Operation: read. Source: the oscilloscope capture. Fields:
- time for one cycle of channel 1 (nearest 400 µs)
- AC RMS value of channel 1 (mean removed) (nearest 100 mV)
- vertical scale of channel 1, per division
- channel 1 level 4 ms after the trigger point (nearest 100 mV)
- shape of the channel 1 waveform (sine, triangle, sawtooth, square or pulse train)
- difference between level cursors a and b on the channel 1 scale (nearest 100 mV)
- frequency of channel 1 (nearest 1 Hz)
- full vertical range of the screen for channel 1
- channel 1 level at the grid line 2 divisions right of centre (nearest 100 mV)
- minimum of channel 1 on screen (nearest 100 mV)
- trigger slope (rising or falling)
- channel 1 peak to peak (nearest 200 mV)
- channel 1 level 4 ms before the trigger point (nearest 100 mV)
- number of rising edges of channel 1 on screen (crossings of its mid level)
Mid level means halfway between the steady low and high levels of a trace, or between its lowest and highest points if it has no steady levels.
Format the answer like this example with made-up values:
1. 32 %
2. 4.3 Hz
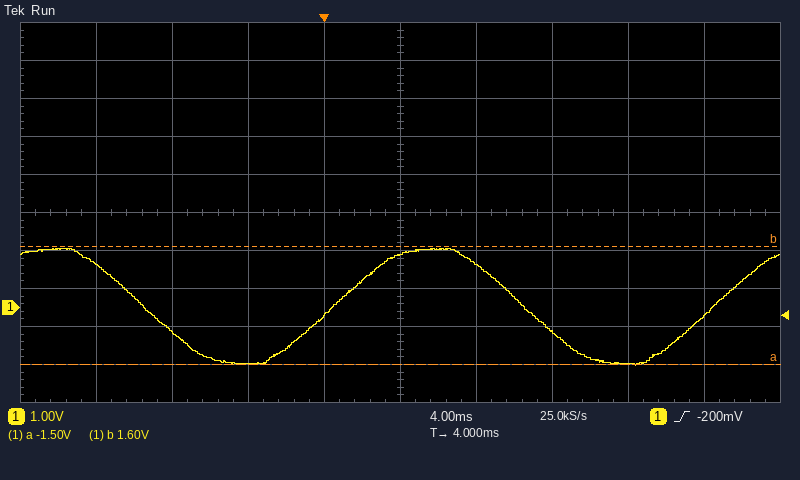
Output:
1. 20.0 ms
2. 1.1 V
3. 1 V
4. 1.4 V
5. sine
6. 3.1 V
7. 50 Hz
8. 10 V
9. -600 mV
10. -1.5 V
11. rising
12. 3.0 V
13. -1.5 V
14. 2
